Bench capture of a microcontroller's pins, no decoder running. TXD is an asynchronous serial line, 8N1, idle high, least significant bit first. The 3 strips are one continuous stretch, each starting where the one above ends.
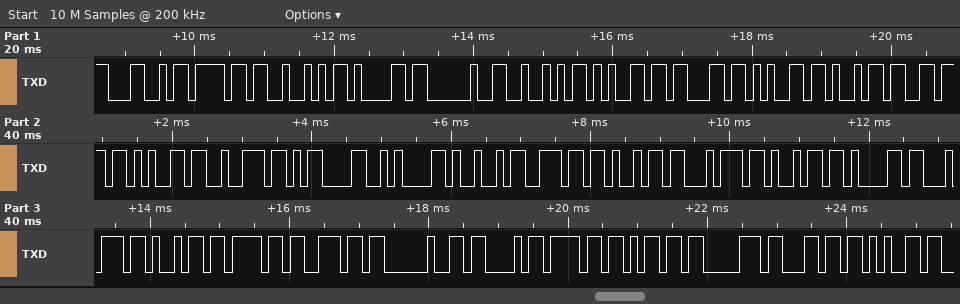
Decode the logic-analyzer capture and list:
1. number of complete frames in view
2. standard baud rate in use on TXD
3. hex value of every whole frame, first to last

32
9600 baud
0x4C 0x6F 0x52 0x61 0x20 0x52 0x65 0x63 0x65 0x69 0x76 0x65 0x72 0x0D 0x0A 0x49 0x6E 0x69 0x74 0x69 0x61 0x74 0x69 0x6F 0x6E 0x20 0x43 0x6F 0x6D 0x70 0x6C 0x65
